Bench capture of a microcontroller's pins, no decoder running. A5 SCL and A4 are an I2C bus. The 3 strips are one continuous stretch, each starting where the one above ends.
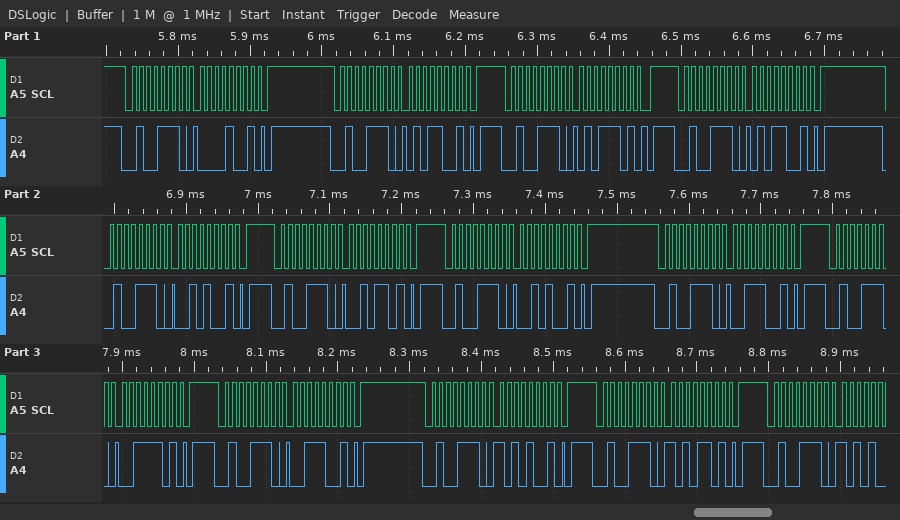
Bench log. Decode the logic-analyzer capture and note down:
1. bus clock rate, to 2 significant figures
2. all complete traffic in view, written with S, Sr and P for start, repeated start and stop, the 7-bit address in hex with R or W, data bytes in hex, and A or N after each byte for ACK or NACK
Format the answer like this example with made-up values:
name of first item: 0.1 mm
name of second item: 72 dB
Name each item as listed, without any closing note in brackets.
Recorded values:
bus clock rate, to 2 significant figures: 100 kHz
all complete traffic in view, written with S, Sr and P for start, repeated start and stop, the 7-bit address in hex with R or W, data bytes in hex, and A or N after each byte for ACK or NACK: S 27W A 09 A P S 27W A 59 A P S 27W A 5D A P S 27W A 59 A P S 27W A 29 A P S 27W A 2D A P S 27W A 29 A P S 27W A 39 A P S 27W A 3D A P S 27W A 39 A P S 27W A A9 A P S 27W A AD A P S 27W A
